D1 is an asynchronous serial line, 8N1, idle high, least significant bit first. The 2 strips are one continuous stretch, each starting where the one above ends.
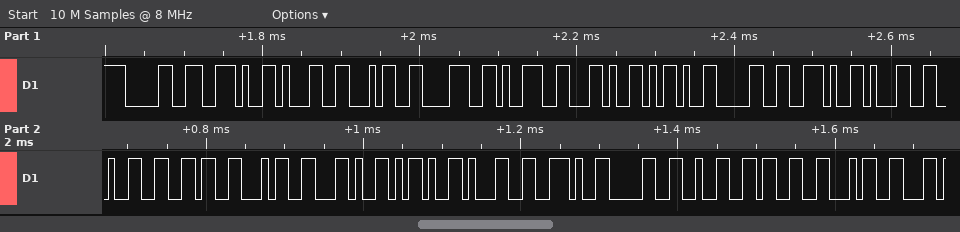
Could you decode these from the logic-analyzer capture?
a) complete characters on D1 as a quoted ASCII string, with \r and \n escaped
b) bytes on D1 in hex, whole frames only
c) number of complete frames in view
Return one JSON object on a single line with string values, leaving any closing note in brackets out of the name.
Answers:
{"complete characters on D1 as a quoted ASCII string, with \\r and \\n escaped": "\"0.1489,-0.1264,-1.0234\"", "bytes on D1 in hex, whole frames only": "0x30 0x2E 0x31 0x34 0x38 0x39 0x2C 0x2D 0x30 0x2E 0x31 0x32 0x36 0x34 0x2C 0x2D 0x31 0x2E 0x30 0x32 0x33 0x34", "number of complete frames in view": "22"}
